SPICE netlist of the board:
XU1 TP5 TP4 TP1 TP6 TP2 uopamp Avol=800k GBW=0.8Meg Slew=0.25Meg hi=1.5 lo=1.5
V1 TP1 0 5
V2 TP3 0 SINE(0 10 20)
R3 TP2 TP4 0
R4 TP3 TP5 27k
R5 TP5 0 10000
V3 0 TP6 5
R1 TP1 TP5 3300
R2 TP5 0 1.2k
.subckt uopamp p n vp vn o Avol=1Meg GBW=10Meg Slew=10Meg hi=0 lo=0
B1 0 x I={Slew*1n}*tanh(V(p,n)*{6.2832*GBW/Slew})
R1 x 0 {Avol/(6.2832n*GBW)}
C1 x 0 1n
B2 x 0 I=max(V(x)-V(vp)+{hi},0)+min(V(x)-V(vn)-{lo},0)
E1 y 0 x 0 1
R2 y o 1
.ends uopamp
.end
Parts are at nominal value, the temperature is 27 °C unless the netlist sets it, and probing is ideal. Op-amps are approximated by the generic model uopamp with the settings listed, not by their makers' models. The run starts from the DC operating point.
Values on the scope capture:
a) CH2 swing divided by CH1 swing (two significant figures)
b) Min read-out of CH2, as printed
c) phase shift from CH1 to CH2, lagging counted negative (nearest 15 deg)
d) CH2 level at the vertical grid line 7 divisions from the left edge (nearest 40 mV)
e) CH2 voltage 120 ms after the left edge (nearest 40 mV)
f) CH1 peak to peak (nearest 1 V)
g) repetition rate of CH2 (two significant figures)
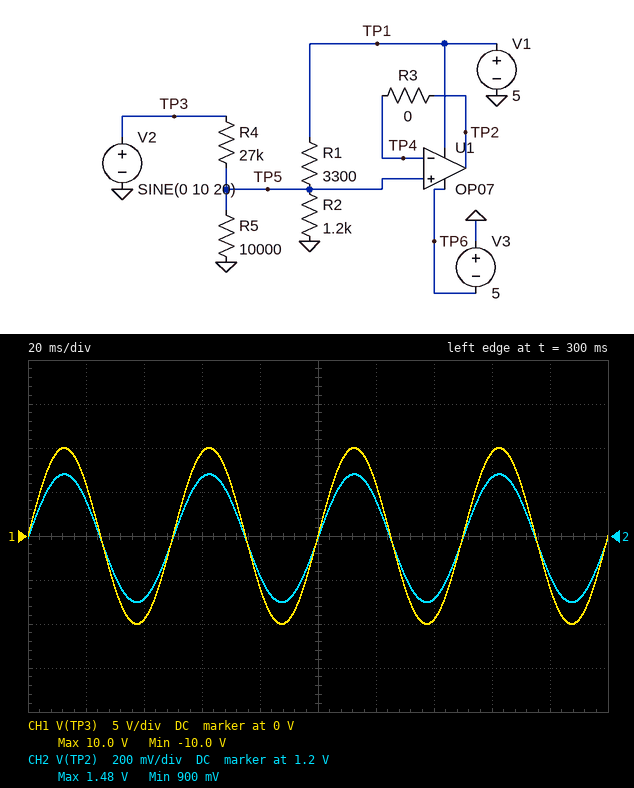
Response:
0.029
900 mV
0 deg
920 mV
1.36 V
20 V
20 Hz
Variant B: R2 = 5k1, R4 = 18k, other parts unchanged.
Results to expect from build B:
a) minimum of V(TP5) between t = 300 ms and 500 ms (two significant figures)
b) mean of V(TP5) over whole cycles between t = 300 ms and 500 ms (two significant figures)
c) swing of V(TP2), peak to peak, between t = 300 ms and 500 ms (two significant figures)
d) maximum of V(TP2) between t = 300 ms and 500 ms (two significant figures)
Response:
1.5 V
2.3 V
1.7 V
3.2 V
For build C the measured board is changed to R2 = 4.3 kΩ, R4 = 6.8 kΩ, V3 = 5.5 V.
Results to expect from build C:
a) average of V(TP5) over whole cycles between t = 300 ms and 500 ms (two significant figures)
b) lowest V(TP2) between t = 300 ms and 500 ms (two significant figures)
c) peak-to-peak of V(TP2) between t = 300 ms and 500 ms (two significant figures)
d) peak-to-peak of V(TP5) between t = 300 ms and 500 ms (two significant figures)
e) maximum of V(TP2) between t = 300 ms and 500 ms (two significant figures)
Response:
1.9 V
57 mV
3.4 V
3.8 V
3.5 V
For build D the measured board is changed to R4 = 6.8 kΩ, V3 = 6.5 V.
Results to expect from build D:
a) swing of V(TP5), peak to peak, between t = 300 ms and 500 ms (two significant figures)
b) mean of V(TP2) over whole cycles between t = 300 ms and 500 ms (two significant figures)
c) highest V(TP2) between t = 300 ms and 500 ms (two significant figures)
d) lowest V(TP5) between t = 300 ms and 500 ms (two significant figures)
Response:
2.1 V
1.1 V
2.2 V
32 mV
